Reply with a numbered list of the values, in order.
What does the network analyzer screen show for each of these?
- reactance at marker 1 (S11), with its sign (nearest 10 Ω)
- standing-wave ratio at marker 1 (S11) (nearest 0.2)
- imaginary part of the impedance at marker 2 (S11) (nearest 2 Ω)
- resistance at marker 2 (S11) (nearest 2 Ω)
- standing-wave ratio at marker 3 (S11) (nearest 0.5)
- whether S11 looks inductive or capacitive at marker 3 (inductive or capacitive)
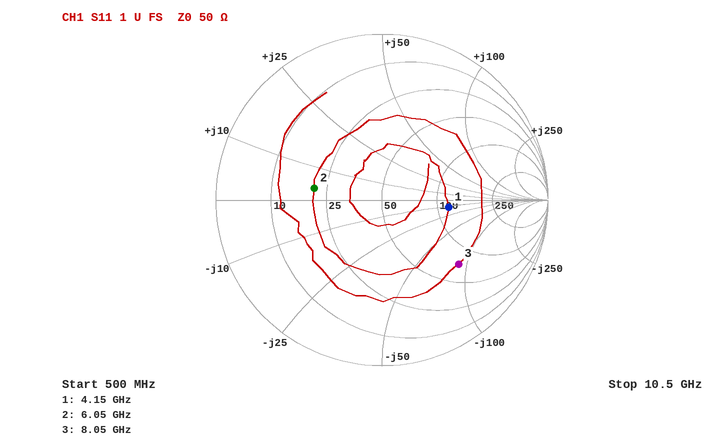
1. -10 Ω
2. 2.4
3. +4 Ω
4. 20 Ω
5. 4.0
6. capacitive
